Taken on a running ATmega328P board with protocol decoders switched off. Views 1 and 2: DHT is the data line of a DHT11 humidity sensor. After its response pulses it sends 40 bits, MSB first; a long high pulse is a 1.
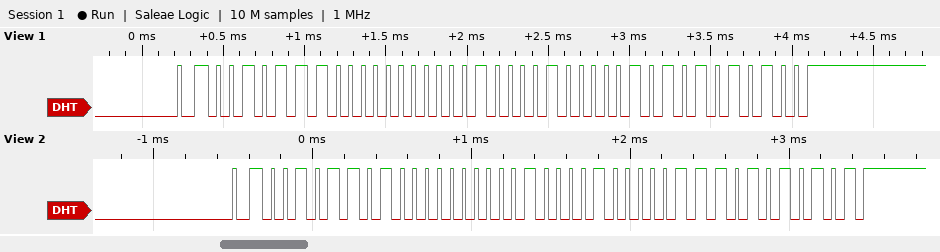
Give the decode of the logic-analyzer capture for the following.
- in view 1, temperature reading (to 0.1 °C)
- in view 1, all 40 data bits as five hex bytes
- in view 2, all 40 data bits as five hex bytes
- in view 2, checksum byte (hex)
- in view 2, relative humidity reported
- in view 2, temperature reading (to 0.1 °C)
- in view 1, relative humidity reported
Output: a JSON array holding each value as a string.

["33.5 °C", "2E 00 21 05 54", "2D 00 21 07 55", "0x55", "45 %", "33.7 °C", "46 %"]
